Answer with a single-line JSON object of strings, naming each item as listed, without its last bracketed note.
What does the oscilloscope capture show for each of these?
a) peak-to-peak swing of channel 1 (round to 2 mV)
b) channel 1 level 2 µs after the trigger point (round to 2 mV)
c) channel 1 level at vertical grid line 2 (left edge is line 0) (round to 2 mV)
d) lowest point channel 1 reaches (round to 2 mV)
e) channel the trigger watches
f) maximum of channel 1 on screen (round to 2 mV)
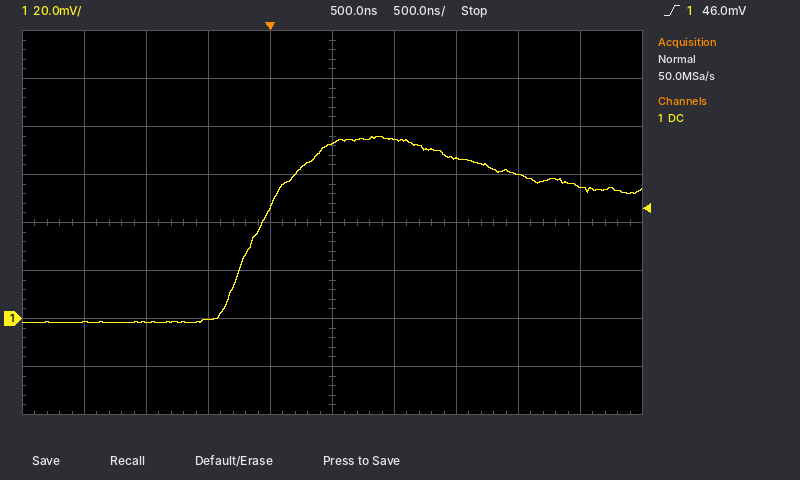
{"peak-to-peak swing of channel 1": "78 mV", "channel 1 level 2 µs after the trigger point": "60 mV", "channel 1 level at vertical grid line 2 (left edge is line 0)": "-2 mV", "lowest point channel 1 reaches": "-2 mV", "channel the trigger watches": "channel 1", "maximum of channel 1 on screen": "76 mV"}
